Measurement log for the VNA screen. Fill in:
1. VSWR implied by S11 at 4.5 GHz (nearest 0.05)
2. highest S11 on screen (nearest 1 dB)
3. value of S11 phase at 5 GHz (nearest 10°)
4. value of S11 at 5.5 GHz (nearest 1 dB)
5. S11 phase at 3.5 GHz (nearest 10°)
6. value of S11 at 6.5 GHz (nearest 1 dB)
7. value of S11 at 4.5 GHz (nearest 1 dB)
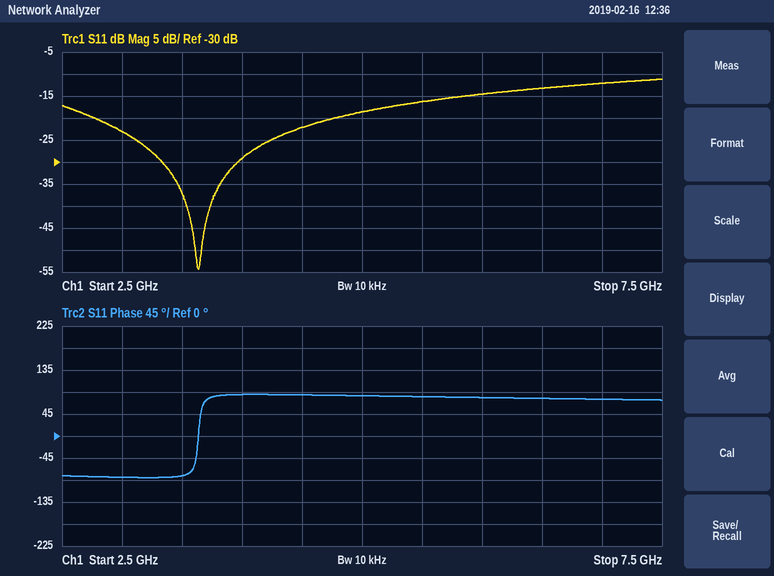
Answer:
1.15
-11 dB
80°
-16 dB
-80°
-13 dB
-22 dB
